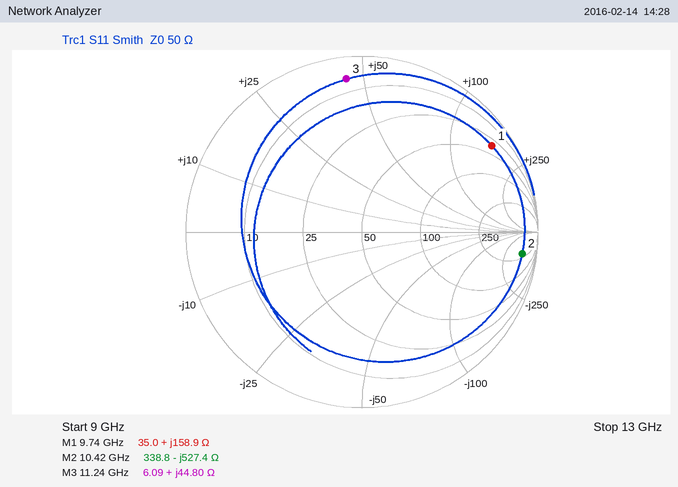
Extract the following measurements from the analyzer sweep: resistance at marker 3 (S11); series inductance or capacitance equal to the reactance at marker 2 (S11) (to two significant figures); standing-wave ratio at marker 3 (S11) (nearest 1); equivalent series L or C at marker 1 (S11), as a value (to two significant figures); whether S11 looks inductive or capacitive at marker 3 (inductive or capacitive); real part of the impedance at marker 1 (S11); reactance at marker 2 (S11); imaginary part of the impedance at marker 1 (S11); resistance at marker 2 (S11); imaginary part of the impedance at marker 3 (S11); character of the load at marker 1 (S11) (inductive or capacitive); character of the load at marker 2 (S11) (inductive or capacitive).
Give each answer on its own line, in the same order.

6.09 Ω
29 fF
15
2.6 nH
inductive
35.0 Ω
-527.4 Ω
+158.9 Ω
338.8 Ω
+44.80 Ω
inductive
capacitive
